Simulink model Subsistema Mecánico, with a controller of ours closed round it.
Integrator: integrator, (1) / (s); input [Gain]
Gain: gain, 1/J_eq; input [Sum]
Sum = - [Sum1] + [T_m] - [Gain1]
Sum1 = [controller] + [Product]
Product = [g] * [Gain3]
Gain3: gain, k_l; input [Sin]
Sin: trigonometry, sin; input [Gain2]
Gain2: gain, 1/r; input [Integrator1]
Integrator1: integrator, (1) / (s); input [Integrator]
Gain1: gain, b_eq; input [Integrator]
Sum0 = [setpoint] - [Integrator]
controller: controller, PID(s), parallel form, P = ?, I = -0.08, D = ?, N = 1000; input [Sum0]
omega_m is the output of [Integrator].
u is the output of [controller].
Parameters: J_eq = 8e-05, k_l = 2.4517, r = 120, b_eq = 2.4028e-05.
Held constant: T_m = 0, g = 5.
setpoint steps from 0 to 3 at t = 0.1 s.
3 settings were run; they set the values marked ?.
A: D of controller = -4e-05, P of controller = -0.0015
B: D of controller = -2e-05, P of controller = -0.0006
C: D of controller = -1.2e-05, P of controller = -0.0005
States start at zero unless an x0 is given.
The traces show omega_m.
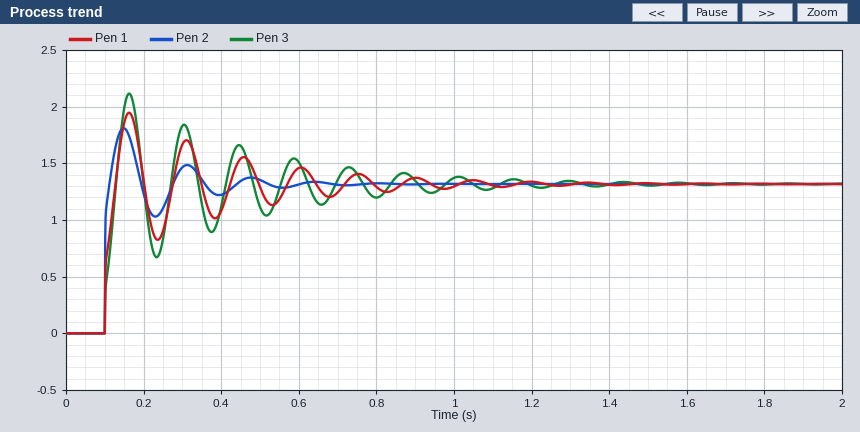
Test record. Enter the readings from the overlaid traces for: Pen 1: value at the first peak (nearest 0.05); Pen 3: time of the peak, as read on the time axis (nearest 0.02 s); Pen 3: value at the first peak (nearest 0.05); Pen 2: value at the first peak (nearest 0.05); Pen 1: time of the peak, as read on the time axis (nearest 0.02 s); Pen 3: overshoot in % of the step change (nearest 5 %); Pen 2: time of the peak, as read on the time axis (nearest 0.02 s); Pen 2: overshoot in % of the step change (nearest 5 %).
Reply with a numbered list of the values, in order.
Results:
1. 1.95
2. 0.16 s
3. 2.10
4. 1.80
5. 0.16 s
6. 60 %
7. 0.14 s
8. 35 %
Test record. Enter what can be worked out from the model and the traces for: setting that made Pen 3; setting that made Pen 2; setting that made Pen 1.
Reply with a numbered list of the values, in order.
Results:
1. C
2. A
3. B
